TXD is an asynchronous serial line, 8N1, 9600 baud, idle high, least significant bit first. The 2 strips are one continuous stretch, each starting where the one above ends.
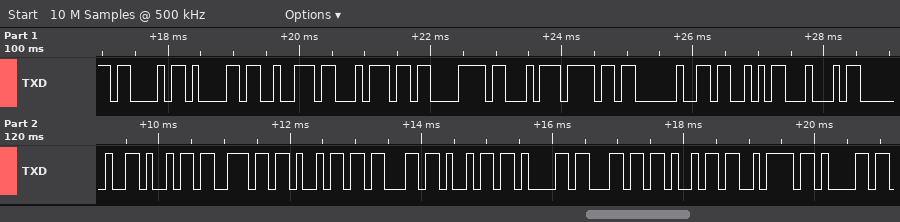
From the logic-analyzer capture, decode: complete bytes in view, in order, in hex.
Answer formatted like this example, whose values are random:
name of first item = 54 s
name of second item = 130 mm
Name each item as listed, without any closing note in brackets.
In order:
complete bytes in view, in order, in hex = 43 61 72 74 C3 A3 6F 20 53 44 20 69 6E 69 63 69 61 6C 69 7A 61
